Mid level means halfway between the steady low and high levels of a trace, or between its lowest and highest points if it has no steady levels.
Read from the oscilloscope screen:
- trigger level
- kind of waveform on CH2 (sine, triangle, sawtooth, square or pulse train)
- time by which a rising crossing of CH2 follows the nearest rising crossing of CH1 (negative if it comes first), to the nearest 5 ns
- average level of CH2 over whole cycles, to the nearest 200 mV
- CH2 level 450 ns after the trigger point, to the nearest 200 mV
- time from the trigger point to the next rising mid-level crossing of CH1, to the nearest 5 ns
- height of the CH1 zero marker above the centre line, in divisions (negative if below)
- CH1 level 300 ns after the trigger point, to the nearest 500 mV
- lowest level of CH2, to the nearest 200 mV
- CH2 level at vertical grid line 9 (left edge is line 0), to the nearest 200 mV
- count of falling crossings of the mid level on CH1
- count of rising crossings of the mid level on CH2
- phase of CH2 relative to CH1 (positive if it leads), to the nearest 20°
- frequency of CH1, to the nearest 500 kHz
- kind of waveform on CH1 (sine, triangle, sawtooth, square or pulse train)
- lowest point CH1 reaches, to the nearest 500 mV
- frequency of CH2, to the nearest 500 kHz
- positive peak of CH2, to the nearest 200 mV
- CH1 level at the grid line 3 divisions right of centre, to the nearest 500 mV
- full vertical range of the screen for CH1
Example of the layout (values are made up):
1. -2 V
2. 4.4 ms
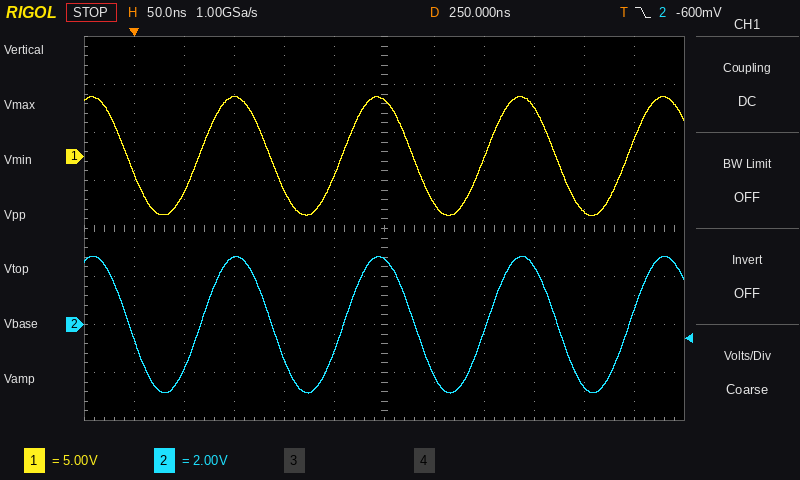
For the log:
1. -600 mV
2. sine
3. 0 ns
4. 0.0 V
5. -2.6 V
6. 65 ns
7. +1.5 div
8. -5.0 V
9. -2.8 V
10. 2.4 V
11. 4
12. 4
13. 0°
14. 7.0 MHz
15. sine
16. -6.0 V
17. 7.0 MHz
18. 2.8 V
19. 5.0 V
20. 40 V
